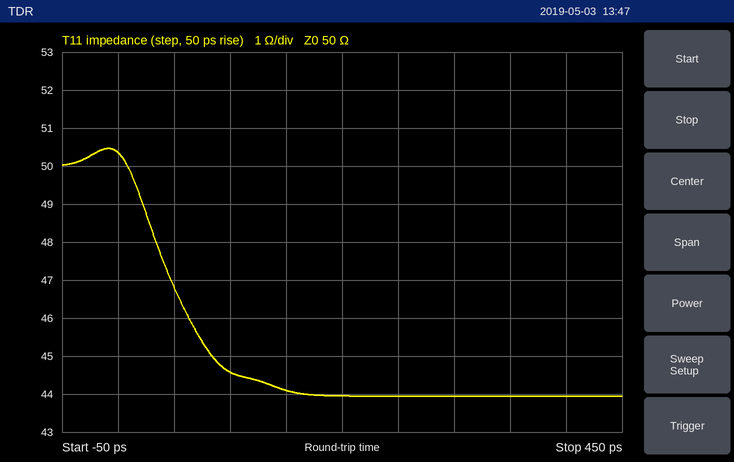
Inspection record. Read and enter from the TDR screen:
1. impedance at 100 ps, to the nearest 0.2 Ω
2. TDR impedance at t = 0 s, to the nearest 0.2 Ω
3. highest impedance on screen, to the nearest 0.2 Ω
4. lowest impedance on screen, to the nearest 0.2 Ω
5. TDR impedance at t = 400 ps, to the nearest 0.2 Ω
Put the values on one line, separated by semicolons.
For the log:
44.6 Ω; 50.4 Ω; 50.4 Ω; 44.0 Ω; 44.0 Ω
